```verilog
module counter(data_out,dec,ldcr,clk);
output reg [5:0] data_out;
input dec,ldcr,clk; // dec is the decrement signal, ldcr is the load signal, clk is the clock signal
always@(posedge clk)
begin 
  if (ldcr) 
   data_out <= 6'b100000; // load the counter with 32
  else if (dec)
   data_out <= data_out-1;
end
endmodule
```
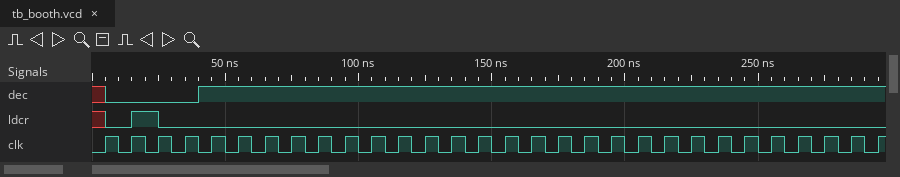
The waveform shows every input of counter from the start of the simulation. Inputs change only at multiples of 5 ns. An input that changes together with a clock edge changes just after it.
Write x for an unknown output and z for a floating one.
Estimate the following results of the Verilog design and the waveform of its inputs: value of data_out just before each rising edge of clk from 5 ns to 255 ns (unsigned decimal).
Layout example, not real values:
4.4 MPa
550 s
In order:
x, x, x, 32, 32, 31, 30, 29, 28, 27, 26, 25, 24, 23, 22, 21, 20, 19, 18, 17, 16, 15, 14, 13, 12, 11
